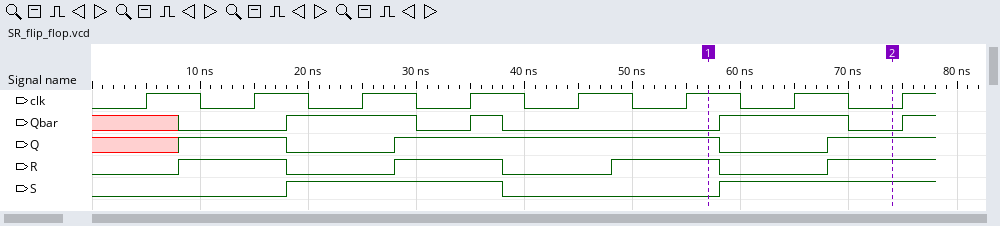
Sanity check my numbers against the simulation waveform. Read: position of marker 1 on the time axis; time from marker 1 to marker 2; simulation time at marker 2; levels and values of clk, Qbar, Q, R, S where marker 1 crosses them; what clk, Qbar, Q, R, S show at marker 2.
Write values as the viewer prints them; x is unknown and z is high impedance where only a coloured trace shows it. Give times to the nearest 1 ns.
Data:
57 ns
17 ns
74 ns
clk=1, Qbar=0, Q=1, R=1, S=0
clk=0, Qbar=0, Q=1, R=1, S=1
